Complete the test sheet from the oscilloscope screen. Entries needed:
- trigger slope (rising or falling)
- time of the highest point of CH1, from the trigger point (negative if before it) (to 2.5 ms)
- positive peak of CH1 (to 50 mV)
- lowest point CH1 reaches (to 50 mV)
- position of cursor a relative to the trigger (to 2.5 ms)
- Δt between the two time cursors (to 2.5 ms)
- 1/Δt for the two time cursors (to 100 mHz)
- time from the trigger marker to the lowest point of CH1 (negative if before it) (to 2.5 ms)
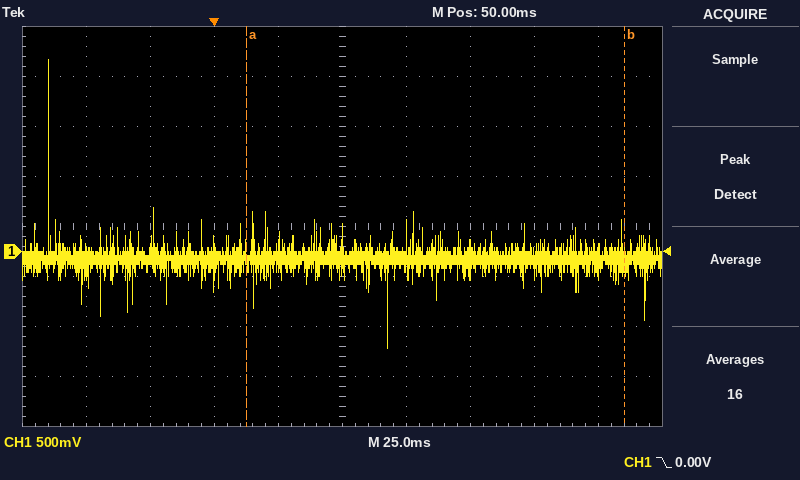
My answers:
falling
-65.0 ms
1.90 V
-950 mV
+12.5 ms
147.5 ms
6.8 Hz
+67.5 ms
